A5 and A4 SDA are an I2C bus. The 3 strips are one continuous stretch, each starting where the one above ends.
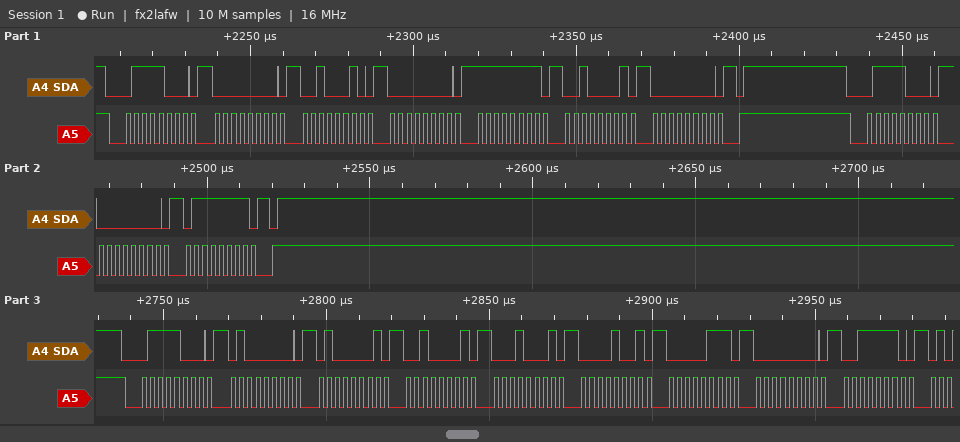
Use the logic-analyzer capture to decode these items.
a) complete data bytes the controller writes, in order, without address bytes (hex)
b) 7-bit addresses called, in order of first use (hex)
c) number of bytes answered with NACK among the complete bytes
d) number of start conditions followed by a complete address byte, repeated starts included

00 22 00 FF 21 00 00 7F 40 41 21 11 09 07 00 3E
0x3C
0
3
